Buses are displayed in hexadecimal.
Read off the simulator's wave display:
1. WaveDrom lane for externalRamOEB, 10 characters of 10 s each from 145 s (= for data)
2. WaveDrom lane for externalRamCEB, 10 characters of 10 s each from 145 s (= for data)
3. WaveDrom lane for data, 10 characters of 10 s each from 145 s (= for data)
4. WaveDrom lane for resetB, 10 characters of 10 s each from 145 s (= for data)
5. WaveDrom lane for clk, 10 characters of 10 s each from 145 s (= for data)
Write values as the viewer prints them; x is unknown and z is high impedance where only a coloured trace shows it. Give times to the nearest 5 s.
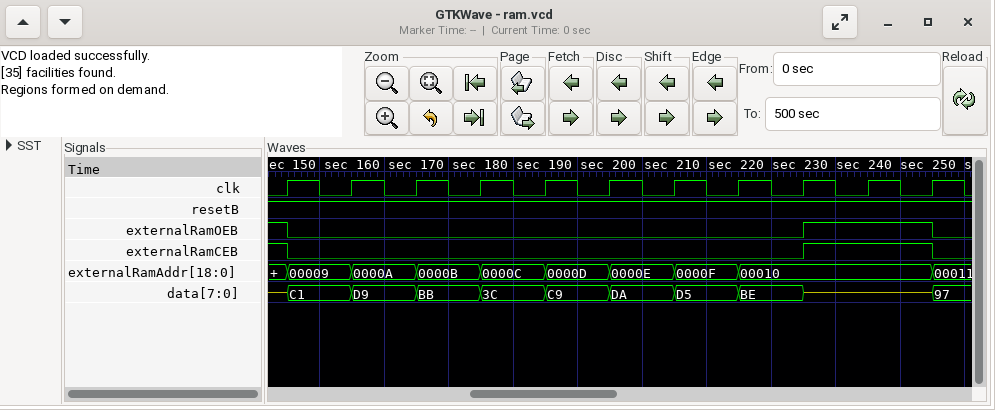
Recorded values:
{name: 'externalRamOEB', wave: '0.......1.'}
{name: 'externalRamCEB', wave: '0.......1.'}
{name: 'data', wave: '========z.', data: 'C1 D9 BB 3C C9 DA D5 BE'}
{name: 'resetB', wave: '1.........'}
{name: 'clk', wave: 'p.........'}
